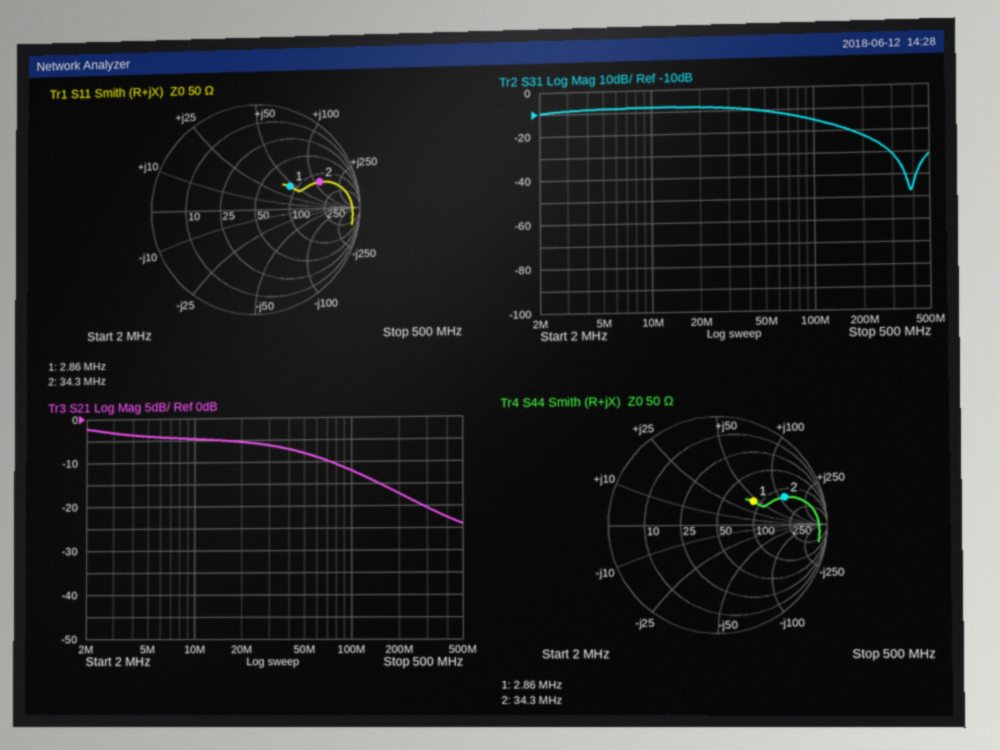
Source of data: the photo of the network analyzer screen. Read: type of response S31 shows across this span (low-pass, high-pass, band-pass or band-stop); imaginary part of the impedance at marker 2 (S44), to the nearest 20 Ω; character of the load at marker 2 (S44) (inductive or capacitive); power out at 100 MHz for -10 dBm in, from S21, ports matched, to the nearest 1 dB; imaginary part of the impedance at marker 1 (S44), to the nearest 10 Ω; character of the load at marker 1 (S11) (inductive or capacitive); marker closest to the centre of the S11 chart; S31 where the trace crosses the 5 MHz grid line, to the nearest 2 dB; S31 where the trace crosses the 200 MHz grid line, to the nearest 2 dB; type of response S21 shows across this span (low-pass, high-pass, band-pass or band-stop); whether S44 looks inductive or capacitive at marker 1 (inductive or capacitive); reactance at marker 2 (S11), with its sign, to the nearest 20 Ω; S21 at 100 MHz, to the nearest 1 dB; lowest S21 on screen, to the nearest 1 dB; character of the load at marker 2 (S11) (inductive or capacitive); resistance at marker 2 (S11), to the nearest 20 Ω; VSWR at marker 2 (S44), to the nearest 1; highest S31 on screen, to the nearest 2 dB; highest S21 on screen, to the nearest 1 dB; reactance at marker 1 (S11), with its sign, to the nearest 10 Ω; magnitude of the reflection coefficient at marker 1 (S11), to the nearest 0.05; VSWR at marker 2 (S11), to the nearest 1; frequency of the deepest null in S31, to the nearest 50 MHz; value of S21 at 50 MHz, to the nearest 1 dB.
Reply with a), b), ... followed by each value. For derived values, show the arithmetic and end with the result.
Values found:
a) low-pass
b) +120 Ω
c) inductive
d) -10 dBm + (-12 dB) = -22 dBm
e) +40 Ω
f) inductive
g) marker 1
h) -8 dB
i) -22 dB
j) low-pass
k) inductive
l) +120 Ω
m) -12 dB
n) -24 dB
o) inductive
p) 140 Ω
q) 5
r) -8 dB
s) -2 dB
t) +40 Ω
u) 0.40
v) 5
w) 400 MHz
x) -8 dB
